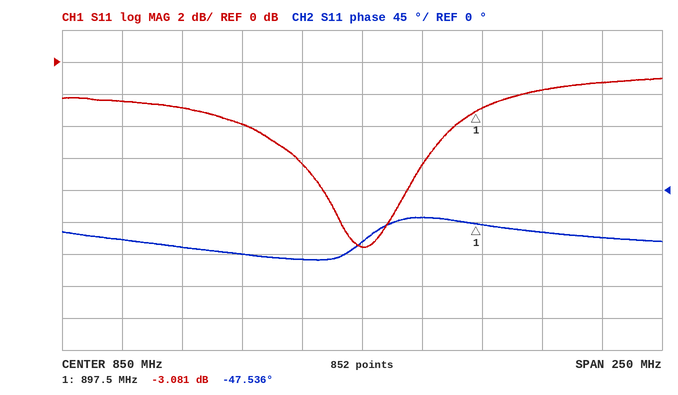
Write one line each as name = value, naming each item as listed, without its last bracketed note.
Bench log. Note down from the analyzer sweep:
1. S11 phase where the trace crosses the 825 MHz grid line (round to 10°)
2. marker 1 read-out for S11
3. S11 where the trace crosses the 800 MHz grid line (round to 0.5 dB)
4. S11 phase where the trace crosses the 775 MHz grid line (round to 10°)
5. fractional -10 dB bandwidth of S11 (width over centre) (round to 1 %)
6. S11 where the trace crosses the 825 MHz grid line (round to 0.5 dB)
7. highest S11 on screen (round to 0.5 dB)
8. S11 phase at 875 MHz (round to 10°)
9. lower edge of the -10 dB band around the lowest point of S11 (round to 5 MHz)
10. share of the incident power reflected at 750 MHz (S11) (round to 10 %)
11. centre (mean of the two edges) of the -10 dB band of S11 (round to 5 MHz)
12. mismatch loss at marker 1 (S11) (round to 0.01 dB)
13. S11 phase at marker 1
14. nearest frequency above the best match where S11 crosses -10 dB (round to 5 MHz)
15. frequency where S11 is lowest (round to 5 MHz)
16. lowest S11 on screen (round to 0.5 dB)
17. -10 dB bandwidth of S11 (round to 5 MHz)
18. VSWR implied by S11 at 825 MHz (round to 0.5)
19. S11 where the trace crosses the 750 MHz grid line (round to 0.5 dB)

S11 phase where the trace crosses the 825 MHz grid line = -100°
marker 1 read-out for S11 = -3.081 dB
S11 where the trace crosses the 800 MHz grid line = -4.0 dB
S11 phase where the trace crosses the 775 MHz grid line = -80°
fractional -10 dB bandwidth of S11 (width over centre) = 2 %
S11 where the trace crosses the 825 MHz grid line = -6.5 dB
highest S11 on screen = -1.0 dB
S11 phase at 875 MHz = -40°
lower edge of the -10 dB band around the lowest point of S11 = 840 MHz
share of the incident power reflected at 750 MHz (S11) = 60 %
centre (mean of the two edges) of the -10 dB band of S11 = 850 MHz
mismatch loss at marker 1 (S11) = 2.94 dB
S11 phase at marker 1 = -47.536°
nearest frequency above the best match where S11 crosses -10 dB = 860 MHz
frequency where S11 is lowest = 850 MHz
lowest S11 on screen = -11.5 dB
-10 dB bandwidth of S11 = 20 MHz
VSWR implied by S11 at 825 MHz = 3.0
S11 where the trace crosses the 750 MHz grid line = -2.5 dB
